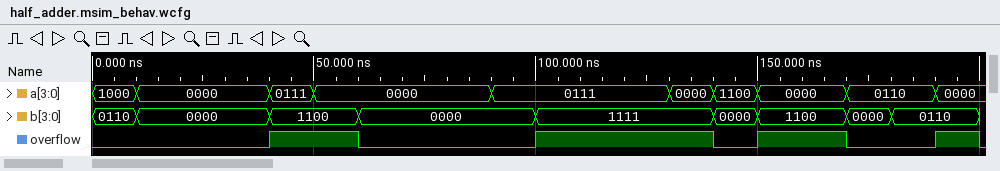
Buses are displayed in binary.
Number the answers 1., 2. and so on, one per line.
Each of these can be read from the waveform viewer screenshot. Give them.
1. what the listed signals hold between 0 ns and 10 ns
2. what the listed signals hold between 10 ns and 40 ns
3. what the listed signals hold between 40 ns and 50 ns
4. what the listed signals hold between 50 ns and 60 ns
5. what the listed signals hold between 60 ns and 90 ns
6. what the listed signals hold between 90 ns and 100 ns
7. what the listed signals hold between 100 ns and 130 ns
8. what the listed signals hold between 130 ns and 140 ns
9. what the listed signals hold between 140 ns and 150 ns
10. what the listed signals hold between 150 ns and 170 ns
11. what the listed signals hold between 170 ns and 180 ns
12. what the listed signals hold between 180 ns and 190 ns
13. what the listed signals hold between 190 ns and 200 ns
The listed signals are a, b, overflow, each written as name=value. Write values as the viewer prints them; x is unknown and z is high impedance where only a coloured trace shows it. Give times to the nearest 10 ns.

1. a=1000, b=0110, overflow=0
2. a=0000, b=0000, overflow=0
3. a=0111, b=1100, overflow=1
4. a=0000, b=1100, overflow=1
5. a=0000, b=0000, overflow=0
6. a=0111, b=0000, overflow=0
7. a=0111, b=1111, overflow=1
8. a=0000, b=1111, overflow=1
9. a=1100, b=0000, overflow=0
10. a=0000, b=1100, overflow=1
11. a=0110, b=0000, overflow=0
12. a=0110, b=0110, overflow=0
13. a=0000, b=0110, overflow=1
